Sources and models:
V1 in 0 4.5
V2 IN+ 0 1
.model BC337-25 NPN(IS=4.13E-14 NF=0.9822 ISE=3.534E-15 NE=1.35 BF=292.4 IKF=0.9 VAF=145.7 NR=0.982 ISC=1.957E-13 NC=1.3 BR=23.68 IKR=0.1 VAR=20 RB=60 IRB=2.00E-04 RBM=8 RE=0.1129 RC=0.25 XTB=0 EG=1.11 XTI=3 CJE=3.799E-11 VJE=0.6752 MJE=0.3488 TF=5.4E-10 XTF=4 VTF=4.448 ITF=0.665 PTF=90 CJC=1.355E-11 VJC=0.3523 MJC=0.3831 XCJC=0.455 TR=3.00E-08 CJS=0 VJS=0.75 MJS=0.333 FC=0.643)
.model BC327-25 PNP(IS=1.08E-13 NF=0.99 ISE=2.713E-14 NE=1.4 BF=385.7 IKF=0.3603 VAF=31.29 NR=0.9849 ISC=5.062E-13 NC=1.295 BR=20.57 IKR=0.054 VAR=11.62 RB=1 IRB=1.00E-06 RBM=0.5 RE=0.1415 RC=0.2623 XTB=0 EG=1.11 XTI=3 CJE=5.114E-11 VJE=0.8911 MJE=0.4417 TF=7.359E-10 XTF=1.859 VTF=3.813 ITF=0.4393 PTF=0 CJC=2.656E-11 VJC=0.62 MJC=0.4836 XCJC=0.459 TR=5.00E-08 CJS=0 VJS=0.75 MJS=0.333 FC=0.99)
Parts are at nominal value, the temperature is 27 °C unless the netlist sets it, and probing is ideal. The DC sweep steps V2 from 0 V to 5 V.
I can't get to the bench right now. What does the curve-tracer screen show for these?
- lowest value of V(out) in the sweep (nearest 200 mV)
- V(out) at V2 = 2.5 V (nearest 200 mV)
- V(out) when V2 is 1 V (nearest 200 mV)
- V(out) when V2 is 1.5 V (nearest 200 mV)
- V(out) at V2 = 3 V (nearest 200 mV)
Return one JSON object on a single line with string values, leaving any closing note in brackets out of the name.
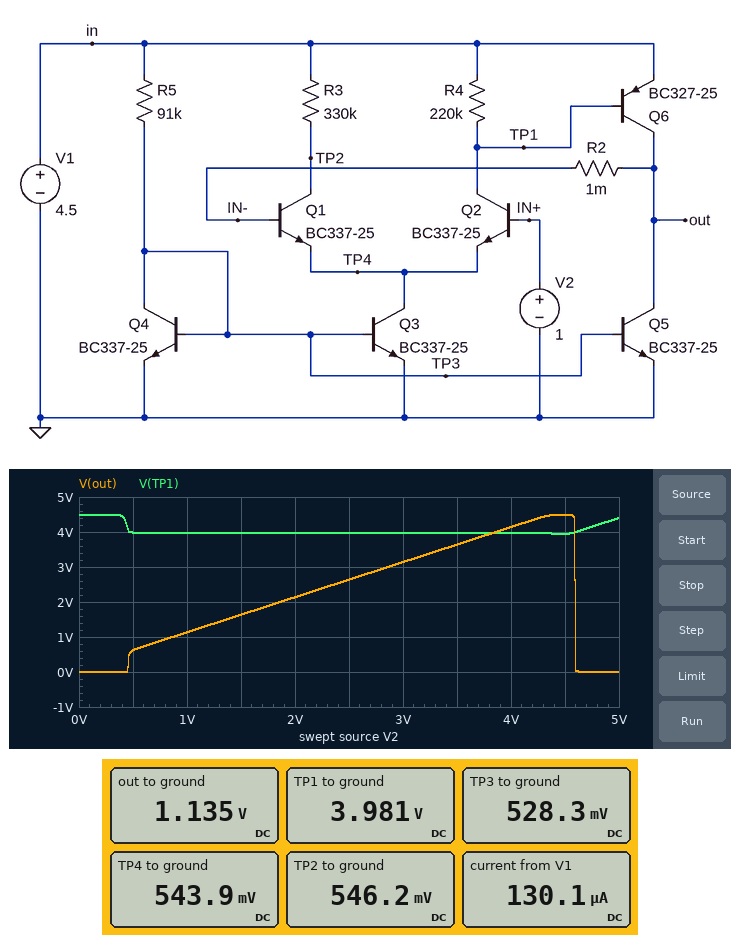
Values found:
{"lowest value of V(out) in the sweep": "0 V", "V(out) at V2 = 2.5 V": "2.6 V", "V(out) when V2 is 1 V": "1.2 V", "V(out) when V2 is 1.5 V": "1.6 V", "V(out) at V2 = 3 V": "3.2 V"}
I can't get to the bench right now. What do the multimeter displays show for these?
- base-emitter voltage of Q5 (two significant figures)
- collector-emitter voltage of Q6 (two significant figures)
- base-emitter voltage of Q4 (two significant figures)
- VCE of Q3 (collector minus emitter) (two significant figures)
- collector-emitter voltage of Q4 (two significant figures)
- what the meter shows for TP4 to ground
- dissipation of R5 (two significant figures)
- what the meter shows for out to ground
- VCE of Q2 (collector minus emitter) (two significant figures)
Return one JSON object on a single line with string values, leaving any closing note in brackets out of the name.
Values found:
{"base-emitter voltage of Q5": "530 mV", "collector-emitter voltage of Q6": "-3.4 V", "base-emitter voltage of Q4": "530 mV", "VCE of Q3 (collector minus emitter)": "540 mV", "collector-emitter voltage of Q4": "530 mV", "what the meter shows for TP4 to ground": "543.9 mV", "dissipation of R5": "170 µW", "what the meter shows for out to ground": "1.135 V", "VCE of Q2 (collector minus emitter)": "3.4 V"}
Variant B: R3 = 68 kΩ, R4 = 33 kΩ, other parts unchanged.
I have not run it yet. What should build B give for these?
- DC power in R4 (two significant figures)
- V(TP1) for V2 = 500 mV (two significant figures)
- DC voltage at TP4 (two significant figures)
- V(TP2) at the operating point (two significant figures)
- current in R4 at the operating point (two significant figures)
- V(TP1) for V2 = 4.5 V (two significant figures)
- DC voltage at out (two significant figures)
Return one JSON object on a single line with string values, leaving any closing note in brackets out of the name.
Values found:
{"DC power in R4": "7.8 µW", "V(TP1) for V2 = 500 mV": "4.2 V", "DC voltage at TP4": "500 mV", "V(TP2) at the operating point": "2.6 V", "current in R4 at the operating point": "15 µA", "V(TP1) for V2 = 4.5 V": "4.0 V", "DC voltage at out": "1.0 V"}
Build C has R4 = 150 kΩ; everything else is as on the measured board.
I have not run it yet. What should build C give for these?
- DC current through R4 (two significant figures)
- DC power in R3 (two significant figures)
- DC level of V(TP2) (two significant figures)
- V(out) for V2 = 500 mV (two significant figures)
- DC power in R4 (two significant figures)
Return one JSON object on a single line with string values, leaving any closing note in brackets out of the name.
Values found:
{"DC current through R4": "3.5 µA", "DC power in R3": "48 µW", "DC level of V(TP2)": "540 mV", "V(out) for V2 = 500 mV": "610 mV", "DC power in R4": "1.8 µW"}
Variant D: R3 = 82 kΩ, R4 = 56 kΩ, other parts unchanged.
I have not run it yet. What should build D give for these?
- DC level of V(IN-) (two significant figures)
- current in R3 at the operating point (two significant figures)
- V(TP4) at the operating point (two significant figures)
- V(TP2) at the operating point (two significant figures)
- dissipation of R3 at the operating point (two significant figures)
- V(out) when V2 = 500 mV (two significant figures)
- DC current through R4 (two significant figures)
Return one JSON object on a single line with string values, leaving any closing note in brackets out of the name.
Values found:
{"DC level of V(IN-)": "1.0 V", "current in R3 at the operating point": "34 µA", "V(TP4) at the operating point": "510 mV", "V(TP2) at the operating point": "1.7 V", "dissipation of R3 at the operating point": "94 µW", "V(out) when V2 = 500 mV": "480 mV", "DC current through R4": "9.0 µA"}
